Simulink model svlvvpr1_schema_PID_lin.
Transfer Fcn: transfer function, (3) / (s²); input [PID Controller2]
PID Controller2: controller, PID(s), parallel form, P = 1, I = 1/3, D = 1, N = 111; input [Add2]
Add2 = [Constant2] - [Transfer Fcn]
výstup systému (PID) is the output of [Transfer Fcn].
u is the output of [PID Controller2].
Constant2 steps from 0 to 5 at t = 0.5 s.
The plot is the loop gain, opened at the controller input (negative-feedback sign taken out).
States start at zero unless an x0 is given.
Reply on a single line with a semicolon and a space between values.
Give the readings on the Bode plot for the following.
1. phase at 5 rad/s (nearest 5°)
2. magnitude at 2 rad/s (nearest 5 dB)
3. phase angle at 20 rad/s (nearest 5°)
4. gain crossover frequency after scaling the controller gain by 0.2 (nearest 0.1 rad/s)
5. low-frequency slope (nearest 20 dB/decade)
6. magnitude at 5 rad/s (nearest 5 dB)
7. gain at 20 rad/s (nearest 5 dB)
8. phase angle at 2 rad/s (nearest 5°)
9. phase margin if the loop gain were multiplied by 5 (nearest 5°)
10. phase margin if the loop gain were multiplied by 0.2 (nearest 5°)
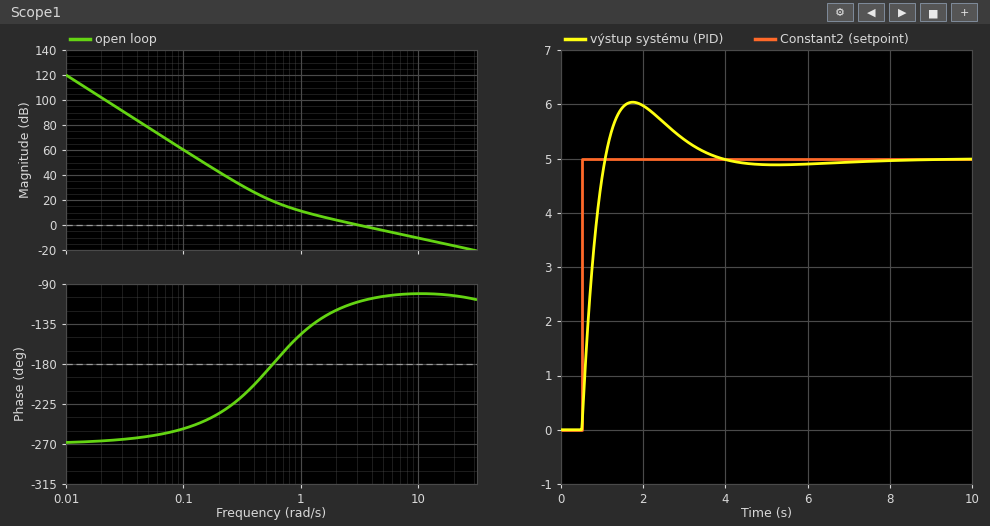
-105°; 5 dB; -105°; 0.8 rad/s; -60 dB/decade; -5 dB; -15 dB; -120°; 80°; 20°
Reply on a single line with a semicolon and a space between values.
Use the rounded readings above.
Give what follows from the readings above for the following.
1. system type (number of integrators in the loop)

3
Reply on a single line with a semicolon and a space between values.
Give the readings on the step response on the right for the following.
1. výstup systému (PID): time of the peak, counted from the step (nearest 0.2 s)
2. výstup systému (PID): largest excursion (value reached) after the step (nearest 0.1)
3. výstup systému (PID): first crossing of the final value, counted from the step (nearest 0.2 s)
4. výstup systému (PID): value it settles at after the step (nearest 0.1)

1.2 s; 6.0; 0.6 s; 5.0
